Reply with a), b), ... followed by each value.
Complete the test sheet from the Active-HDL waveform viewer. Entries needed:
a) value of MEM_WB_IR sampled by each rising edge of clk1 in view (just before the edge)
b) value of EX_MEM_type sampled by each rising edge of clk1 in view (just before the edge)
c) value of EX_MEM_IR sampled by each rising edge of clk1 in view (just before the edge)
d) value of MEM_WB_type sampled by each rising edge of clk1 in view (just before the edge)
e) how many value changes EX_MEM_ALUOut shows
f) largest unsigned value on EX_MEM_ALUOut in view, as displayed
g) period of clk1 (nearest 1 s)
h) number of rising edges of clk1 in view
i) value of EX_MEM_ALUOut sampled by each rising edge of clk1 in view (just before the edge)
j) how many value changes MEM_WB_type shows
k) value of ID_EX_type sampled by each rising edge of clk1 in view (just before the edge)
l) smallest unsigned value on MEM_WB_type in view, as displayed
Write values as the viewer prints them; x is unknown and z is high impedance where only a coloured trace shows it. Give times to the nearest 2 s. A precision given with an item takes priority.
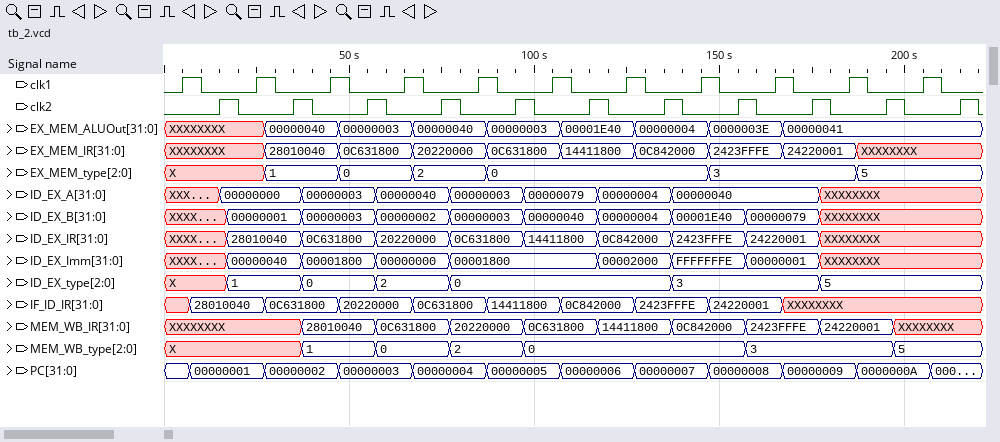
a) XXXXXXXX, XXXXXXXX, 28010040, 0C631800, 20220000, 0C631800, 14411800, 0C842000, 2423FFFE, 24220001, XXXXXXXX
b) X, X, 1, 0, 2, 0, 0, 0, 3, 3, 5
c) XXXXXXXX, XXXXXXXX, 28010040, 0C631800, 20220000, 0C631800, 14411800, 0C842000, 2423FFFE, 24220001, XXXXXXXX
d) X, X, 1, 0, 2, 0, 0, 0, 3, 3, 5
e) 8
f) 00001E40
g) 20 s
h) 11
i) XXXXXXXX, XXXXXXXX, 00000040, 00000003, 00000040, 00000003, 00001E40, 00000004, 0000003E, 00000041, 00000041
j) 6
k) X, 1, 0, 2, 0, 0, 0, 3, 3, 5, 5
l) 0
